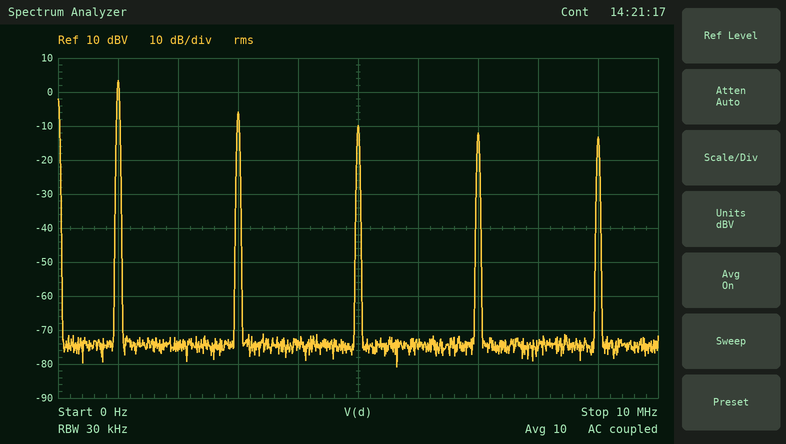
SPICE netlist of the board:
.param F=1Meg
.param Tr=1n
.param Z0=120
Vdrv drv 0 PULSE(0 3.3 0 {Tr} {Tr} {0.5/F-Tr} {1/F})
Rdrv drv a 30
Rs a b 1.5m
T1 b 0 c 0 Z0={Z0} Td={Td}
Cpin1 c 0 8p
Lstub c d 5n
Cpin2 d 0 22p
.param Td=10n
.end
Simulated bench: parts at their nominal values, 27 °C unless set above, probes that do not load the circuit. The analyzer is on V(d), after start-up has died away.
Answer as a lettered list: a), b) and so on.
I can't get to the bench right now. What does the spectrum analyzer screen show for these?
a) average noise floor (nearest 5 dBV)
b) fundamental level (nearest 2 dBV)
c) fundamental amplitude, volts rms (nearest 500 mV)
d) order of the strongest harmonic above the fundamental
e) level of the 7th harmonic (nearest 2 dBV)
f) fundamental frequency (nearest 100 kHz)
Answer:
a) -75 dBV
b) 4 dBV
c) 1.5 V
d) 3
e) -12 dBV
f) 1.0 MHz
